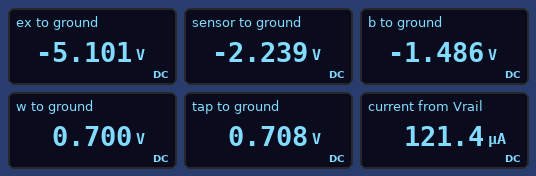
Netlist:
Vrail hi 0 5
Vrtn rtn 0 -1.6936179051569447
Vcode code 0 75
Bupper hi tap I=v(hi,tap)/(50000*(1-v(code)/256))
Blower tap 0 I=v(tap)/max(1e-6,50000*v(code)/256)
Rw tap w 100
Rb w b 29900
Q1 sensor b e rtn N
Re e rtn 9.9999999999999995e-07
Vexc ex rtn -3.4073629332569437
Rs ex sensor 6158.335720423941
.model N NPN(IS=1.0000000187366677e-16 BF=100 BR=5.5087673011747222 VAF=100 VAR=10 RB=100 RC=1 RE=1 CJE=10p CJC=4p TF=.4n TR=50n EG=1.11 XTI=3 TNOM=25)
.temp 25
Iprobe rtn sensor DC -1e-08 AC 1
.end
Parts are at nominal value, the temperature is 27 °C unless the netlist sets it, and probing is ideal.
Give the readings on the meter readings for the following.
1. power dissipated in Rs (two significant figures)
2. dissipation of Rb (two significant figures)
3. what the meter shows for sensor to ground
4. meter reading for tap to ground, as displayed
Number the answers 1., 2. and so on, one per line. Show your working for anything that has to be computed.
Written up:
1. (-2.239 V - (-5.101 V))^2 / 6.158 kΩ = 1.3 mW
2. (700 mV - (-1.486 V))^2 / 29.9 kΩ = 160 µW
3. -2.239 V
4. 0.708 V
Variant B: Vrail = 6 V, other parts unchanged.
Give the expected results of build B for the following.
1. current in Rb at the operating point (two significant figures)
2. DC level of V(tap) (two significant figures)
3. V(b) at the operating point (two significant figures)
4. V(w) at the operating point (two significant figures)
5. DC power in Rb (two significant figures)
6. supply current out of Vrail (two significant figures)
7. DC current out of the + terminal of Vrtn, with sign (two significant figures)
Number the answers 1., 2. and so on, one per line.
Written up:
1. 77 µA
2. 960 mV
3. -1.4 V
4. 950 mV
5. 180 µW
6. 140 µA
7. -77 µA
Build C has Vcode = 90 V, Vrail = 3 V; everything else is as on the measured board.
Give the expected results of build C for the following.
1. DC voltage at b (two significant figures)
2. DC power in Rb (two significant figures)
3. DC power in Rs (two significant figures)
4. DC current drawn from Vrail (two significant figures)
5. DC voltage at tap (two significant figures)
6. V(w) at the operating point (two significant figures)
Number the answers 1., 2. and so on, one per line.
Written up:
1. -1.7 V
2. 130 µW
3. 1.1 mW
4. 83 µA
5. 300 mV
6. 290 mV
